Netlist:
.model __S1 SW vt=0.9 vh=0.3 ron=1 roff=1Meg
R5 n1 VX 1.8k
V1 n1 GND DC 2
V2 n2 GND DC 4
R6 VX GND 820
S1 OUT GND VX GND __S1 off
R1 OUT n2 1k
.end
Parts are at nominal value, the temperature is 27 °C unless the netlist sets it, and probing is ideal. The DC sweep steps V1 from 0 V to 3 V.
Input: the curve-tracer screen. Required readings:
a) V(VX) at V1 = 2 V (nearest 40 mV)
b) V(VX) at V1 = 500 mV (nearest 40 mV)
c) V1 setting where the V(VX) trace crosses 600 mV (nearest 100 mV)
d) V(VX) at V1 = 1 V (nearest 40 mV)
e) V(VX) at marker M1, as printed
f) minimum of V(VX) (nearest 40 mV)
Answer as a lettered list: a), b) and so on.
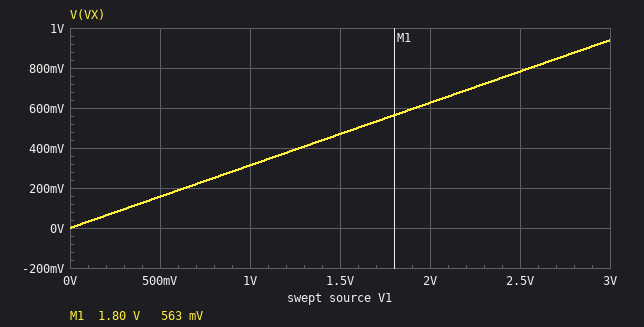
a) 640 mV
b) 160 mV
c) 1.9 V
d) 320 mV
e) 563 mV
f) 0 V
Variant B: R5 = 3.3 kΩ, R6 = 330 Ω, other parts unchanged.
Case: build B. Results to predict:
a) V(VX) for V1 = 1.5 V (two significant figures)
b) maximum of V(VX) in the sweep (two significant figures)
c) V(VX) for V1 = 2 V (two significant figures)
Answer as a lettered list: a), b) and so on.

a) 140 mV
b) 270 mV
c) 180 mV
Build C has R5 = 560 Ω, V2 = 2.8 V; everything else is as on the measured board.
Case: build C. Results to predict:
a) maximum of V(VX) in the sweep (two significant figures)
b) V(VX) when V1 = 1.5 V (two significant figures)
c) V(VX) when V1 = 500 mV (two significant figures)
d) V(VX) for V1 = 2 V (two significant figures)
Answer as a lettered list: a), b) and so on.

a) 1.8 V
b) 890 mV
c) 300 mV
d) 1.2 V
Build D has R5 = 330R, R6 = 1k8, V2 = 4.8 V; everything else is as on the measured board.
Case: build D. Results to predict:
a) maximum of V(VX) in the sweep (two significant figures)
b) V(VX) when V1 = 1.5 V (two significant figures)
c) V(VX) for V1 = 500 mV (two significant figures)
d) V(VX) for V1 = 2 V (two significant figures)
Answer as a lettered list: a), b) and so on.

a) 2.5 V
b) 1.3 V
c) 420 mV
d) 1.7 V
